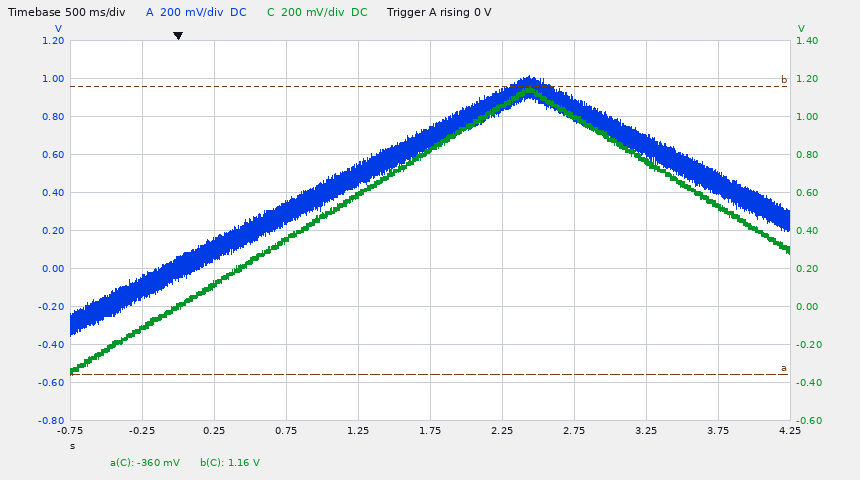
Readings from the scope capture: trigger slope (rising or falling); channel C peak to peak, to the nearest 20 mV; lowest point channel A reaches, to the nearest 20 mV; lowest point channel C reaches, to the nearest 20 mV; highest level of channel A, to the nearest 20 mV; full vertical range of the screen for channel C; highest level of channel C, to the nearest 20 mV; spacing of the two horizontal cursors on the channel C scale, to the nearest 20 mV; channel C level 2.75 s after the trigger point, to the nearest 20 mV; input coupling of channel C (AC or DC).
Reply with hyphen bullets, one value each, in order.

- rising
- 1.52 V
- -360 mV
- -360 mV
- 1.02 V
- 2 V
- 1.16 V
- 1.52 V
- 1.00 V
- DC
